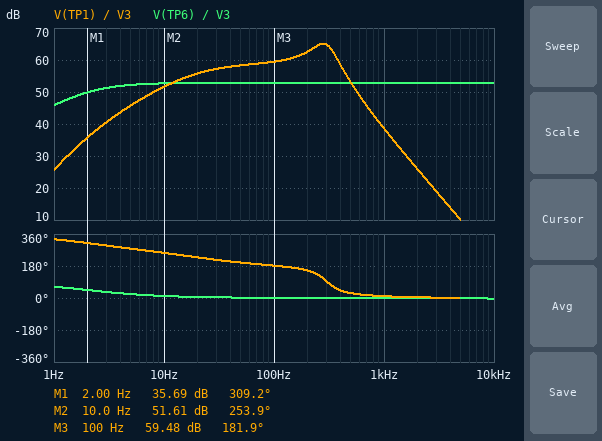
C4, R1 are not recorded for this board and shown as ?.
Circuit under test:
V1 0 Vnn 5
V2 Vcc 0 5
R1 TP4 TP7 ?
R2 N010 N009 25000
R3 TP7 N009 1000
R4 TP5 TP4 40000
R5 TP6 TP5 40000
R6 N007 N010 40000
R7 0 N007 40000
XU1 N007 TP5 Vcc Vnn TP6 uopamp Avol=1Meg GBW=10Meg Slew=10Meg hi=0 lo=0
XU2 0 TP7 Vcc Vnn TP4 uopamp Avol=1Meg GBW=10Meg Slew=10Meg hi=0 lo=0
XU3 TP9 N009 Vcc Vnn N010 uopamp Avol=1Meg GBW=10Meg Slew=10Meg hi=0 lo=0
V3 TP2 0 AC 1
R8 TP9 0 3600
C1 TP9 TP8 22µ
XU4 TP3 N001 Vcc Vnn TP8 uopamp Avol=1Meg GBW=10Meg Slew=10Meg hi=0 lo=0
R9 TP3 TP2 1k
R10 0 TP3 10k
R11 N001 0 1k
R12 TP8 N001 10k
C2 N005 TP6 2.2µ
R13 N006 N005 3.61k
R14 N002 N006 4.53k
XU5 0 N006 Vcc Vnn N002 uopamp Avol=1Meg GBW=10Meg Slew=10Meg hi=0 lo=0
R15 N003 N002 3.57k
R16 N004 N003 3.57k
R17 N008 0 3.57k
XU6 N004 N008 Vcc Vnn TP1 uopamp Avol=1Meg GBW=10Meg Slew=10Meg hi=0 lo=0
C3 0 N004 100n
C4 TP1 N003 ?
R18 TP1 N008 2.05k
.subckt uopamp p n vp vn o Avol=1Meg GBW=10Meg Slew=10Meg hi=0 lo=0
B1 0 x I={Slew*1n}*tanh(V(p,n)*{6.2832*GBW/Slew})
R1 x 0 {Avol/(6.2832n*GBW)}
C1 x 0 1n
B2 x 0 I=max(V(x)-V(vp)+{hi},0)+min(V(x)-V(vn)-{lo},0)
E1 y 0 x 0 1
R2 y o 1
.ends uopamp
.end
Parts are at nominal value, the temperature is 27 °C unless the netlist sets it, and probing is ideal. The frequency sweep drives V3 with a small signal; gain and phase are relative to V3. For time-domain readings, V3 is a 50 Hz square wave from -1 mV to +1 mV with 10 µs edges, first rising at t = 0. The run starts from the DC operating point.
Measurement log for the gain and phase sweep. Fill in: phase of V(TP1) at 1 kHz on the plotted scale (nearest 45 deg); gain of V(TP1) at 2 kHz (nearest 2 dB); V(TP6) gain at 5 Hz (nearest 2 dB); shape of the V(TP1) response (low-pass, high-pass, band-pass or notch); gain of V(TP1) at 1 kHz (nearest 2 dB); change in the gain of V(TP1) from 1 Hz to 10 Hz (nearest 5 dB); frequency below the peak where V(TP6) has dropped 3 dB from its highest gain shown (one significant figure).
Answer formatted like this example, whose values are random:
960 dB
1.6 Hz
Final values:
0 deg
26 dB
52 dB
band-pass
38 dB
25 dB
2 Hz
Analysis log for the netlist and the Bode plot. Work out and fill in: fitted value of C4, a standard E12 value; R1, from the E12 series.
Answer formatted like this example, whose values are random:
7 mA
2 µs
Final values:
220 nF
18 kΩ
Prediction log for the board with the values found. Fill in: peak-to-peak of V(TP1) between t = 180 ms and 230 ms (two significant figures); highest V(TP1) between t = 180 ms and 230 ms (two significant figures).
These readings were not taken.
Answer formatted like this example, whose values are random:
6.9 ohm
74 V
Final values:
3.9 V
2.0 V
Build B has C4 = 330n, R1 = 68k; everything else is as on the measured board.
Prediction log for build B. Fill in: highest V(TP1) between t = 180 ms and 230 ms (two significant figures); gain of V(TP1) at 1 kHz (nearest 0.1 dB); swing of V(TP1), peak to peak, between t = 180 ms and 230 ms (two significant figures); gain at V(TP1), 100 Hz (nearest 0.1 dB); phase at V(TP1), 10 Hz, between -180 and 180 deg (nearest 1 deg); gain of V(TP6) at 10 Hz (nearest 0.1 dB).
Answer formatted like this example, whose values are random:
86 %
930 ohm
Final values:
5.0 V
41.5 dB
10 V
66.8 dB
-105 deg
59.3 dB
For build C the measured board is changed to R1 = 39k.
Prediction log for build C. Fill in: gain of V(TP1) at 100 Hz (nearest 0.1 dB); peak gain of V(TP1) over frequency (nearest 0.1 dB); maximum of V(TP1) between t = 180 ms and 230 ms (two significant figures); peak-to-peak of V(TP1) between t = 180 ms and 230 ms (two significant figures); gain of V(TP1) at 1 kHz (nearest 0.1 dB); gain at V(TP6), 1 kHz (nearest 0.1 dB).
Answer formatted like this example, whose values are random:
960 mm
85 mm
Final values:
62.9 dB
68.5 dB
2.9 V
5.8 V
42.0 dB
56.3 dB
